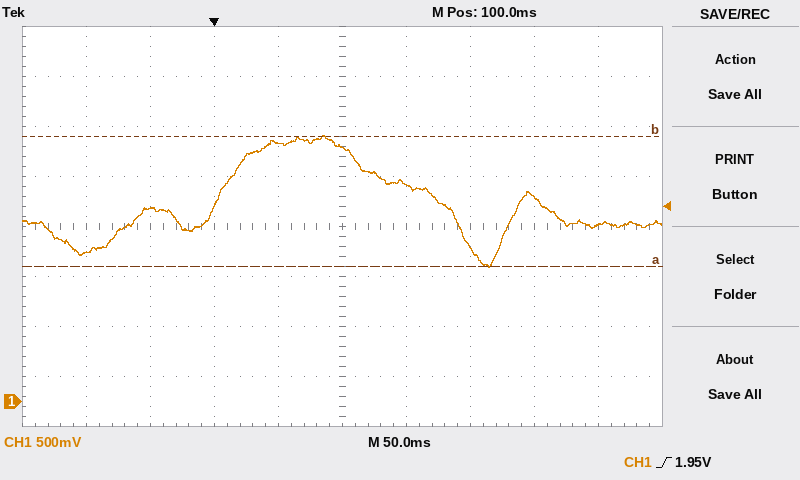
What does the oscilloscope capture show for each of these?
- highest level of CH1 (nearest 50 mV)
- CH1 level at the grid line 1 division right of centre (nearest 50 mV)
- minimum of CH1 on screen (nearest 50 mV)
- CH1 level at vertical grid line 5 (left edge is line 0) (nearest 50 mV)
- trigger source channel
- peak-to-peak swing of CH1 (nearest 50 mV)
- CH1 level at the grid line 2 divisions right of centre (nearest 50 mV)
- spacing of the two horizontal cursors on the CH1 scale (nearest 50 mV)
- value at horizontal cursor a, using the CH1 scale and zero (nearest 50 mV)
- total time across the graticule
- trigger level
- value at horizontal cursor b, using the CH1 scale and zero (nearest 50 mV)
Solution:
2.65 V
2.15 V
1.35 V
2.55 V
CH1
1.30 V
1.55 V
1.30 V
1.35 V
500 ms
1.95 V
2.65 V
